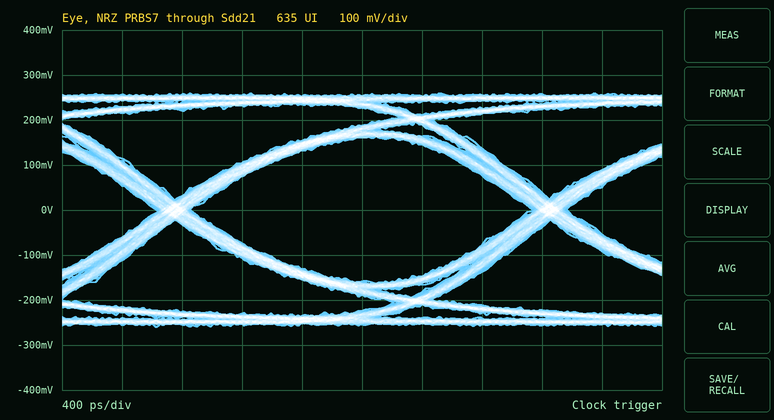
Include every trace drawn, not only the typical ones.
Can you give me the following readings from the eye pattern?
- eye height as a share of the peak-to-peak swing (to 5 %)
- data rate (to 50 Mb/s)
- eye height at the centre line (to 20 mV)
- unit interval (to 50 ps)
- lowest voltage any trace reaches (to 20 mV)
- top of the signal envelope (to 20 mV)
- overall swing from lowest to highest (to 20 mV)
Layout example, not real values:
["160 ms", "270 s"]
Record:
["60 %", "400 Mb/s", "320 mV", "2.50 ns", "-260 mV", "260 mV", "520 mV"]
